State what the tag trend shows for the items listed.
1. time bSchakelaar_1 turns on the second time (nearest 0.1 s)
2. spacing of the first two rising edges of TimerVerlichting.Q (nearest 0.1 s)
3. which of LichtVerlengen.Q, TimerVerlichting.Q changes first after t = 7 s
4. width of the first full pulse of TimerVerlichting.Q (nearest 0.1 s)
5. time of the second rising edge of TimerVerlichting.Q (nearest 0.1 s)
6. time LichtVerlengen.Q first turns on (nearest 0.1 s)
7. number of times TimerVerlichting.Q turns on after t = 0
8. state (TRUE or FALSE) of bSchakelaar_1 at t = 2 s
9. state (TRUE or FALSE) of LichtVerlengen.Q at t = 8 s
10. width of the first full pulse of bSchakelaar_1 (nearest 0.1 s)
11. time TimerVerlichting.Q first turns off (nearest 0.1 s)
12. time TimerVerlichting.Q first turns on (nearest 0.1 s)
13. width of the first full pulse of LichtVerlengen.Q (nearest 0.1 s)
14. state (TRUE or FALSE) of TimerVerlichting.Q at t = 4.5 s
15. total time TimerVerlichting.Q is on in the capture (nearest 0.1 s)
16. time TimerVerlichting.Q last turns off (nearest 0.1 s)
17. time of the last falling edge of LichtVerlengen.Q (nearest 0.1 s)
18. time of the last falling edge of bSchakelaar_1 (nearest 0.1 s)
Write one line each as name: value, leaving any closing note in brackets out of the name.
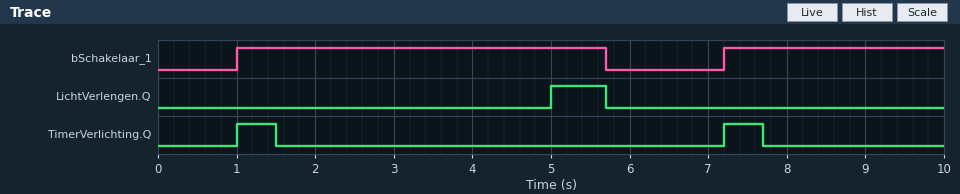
time bSchakelaar_1 turns on the second time: 7.2 s
spacing of the first two rising edges of TimerVerlichting.Q: 6.2 s
which of LichtVerlengen.Q, TimerVerlichting.Q changes first after t = 7 s: TimerVerlichting.Q
width of the first full pulse of TimerVerlichting.Q: 0.5 s
time of the second rising edge of TimerVerlichting.Q: 7.2 s
time LichtVerlengen.Q first turns on: 5.0 s
number of times TimerVerlichting.Q turns on after t = 0: 2
state (TRUE or FALSE) of bSchakelaar_1 at t = 2 s: TRUE
state (TRUE or FALSE) of LichtVerlengen.Q at t = 8 s: FALSE
width of the first full pulse of bSchakelaar_1: 4.7 s
time TimerVerlichting.Q first turns off: 1.5 s
time TimerVerlichting.Q first turns on: 1.0 s
width of the first full pulse of LichtVerlengen.Q: 0.7 s
state (TRUE or FALSE) of TimerVerlichting.Q at t = 4.5 s: FALSE
total time TimerVerlichting.Q is on in the capture: 1.0 s
time TimerVerlichting.Q last turns off: 7.7 s
time of the last falling edge of LichtVerlengen.Q: 5.7 s
time of the last falling edge of bSchakelaar_1: 5.7 s
